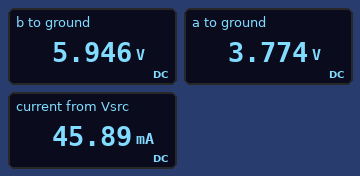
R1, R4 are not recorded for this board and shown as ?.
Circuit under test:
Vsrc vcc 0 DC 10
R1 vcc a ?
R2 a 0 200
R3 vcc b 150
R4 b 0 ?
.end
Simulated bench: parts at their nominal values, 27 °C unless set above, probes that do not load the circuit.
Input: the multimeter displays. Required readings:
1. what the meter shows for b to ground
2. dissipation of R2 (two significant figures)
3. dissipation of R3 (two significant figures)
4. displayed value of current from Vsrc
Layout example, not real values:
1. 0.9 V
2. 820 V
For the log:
1. 5.946 V
2. 71 mW
3. 110 mW
4. 45.89 mA
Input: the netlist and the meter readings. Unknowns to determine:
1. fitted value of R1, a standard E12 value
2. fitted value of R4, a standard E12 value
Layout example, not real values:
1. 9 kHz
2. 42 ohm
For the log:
1. 330 Ω
2. 220 Ω
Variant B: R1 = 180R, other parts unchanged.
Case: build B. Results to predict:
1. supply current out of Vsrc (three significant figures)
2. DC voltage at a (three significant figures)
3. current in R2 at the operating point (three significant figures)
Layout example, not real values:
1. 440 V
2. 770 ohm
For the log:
1. 53.3 mA
2. 5.26 V
3. 26.3 mA
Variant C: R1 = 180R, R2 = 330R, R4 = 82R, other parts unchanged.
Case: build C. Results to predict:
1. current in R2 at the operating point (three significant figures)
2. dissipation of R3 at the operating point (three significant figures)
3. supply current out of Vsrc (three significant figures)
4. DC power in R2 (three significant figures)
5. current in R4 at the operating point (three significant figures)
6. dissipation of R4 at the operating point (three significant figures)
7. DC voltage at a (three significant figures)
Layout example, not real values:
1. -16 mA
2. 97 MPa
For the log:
1. 19.6 mA
2. 279 mW
3. 62.7 mA
4. 127 mW
5. 43.1 mA
6. 152 mW
7. 6.47 V
